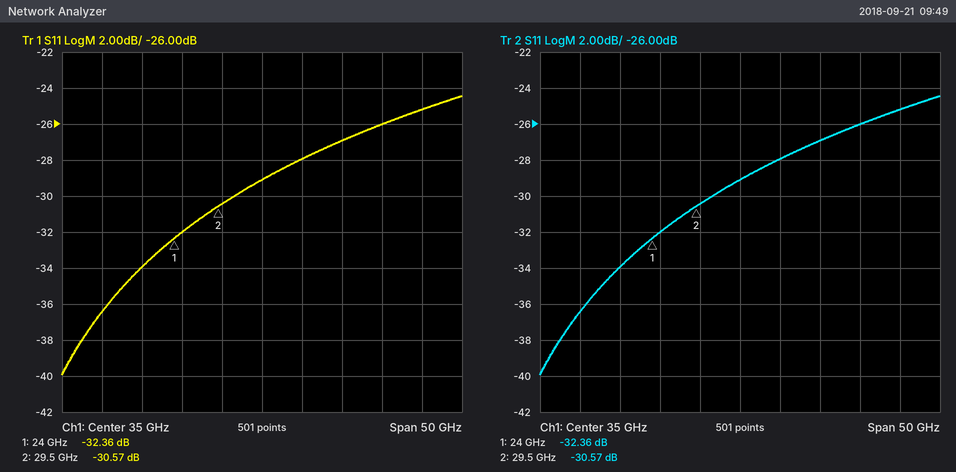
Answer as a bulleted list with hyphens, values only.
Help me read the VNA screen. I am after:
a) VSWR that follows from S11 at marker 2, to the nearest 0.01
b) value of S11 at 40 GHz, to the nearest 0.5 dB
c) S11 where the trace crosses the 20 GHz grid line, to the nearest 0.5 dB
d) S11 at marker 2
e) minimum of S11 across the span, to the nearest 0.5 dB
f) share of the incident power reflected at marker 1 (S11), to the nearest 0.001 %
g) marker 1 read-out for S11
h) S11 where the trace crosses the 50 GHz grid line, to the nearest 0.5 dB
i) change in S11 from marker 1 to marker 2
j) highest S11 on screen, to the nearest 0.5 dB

- 1.06
- -28.0 dB
- -34.0 dB
- -30.57 dB
- -40.0 dB
- 0.058 %
- -32.36 dB
- -26.0 dB
- 1.79 dB
- -24.5 dB
